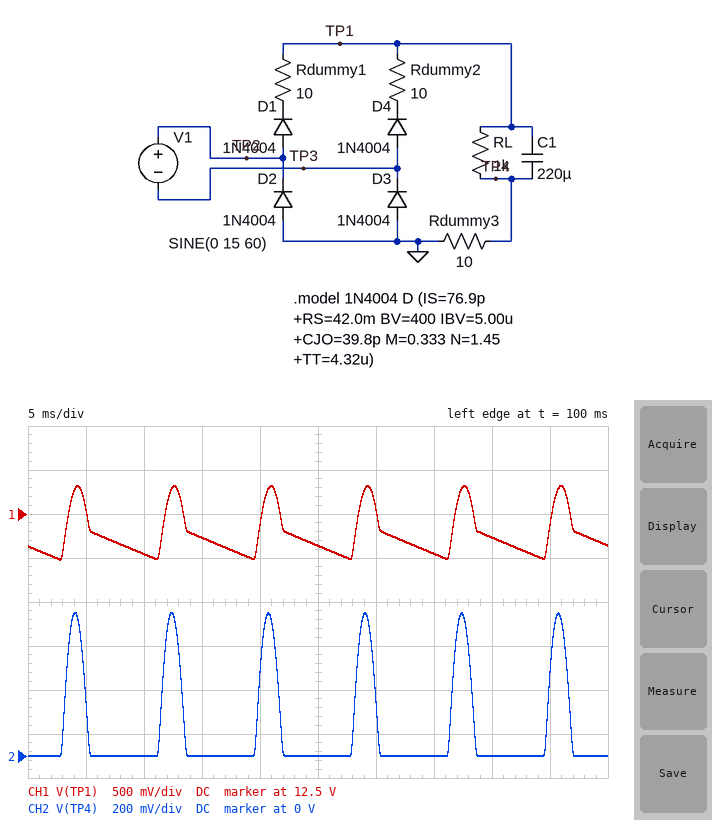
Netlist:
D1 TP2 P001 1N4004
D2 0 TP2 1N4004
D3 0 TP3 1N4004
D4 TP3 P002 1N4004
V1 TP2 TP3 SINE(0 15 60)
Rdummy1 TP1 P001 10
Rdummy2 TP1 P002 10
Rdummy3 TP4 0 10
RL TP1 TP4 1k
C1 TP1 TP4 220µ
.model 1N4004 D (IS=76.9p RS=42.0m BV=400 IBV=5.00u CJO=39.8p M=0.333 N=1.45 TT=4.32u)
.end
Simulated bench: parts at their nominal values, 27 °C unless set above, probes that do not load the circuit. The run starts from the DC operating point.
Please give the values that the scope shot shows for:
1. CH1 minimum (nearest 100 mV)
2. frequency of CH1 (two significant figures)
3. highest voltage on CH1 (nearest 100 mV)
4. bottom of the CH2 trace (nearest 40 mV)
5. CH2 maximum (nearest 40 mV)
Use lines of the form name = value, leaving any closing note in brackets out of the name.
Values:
CH1 minimum = 12.0 V
frequency of CH1 = 120 Hz
highest voltage on CH1 = 12.8 V
bottom of the CH2 trace = 0 V
CH2 maximum = 640 mV
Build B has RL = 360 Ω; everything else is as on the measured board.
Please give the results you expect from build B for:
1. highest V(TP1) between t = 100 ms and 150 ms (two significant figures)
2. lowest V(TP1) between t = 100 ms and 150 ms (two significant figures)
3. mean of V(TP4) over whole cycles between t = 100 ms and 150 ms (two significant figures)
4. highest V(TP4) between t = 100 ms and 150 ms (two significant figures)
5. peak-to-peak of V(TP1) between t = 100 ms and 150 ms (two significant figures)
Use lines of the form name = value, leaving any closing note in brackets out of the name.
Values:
highest V(TP1) between t = 100 ms and 150 ms = 12 V
lowest V(TP1) between t = 100 ms and 150 ms = 11 V
mean of V(TP4) over whole cycles between t = 100 ms and 150 ms = 300 mV
highest V(TP4) between t = 100 ms and 150 ms = 1.2 V
peak-to-peak of V(TP1) between t = 100 ms and 150 ms = 1.6 V
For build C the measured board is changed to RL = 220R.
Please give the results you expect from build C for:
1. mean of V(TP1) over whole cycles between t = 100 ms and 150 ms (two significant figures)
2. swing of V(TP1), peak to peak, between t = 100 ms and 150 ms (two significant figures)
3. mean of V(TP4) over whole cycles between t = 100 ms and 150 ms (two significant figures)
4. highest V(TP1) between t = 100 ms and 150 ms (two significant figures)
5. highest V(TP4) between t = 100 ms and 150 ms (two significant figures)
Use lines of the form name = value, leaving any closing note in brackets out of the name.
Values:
mean of V(TP1) over whole cycles between t = 100 ms and 150 ms = 11 V
swing of V(TP1), peak to peak, between t = 100 ms and 150 ms = 2.2 V
mean of V(TP4) over whole cycles between t = 100 ms and 150 ms = 460 mV
highest V(TP1) between t = 100 ms and 150 ms = 12 V
highest V(TP4) between t = 100 ms and 150 ms = 1.6 V
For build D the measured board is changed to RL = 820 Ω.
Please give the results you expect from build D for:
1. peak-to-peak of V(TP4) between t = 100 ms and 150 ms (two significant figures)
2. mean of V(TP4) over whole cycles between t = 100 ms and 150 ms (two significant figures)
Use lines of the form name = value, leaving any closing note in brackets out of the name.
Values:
peak-to-peak of V(TP4) between t = 100 ms and 150 ms = 740 mV
mean of V(TP4) over whole cycles between t = 100 ms and 150 ms = 150 mV
